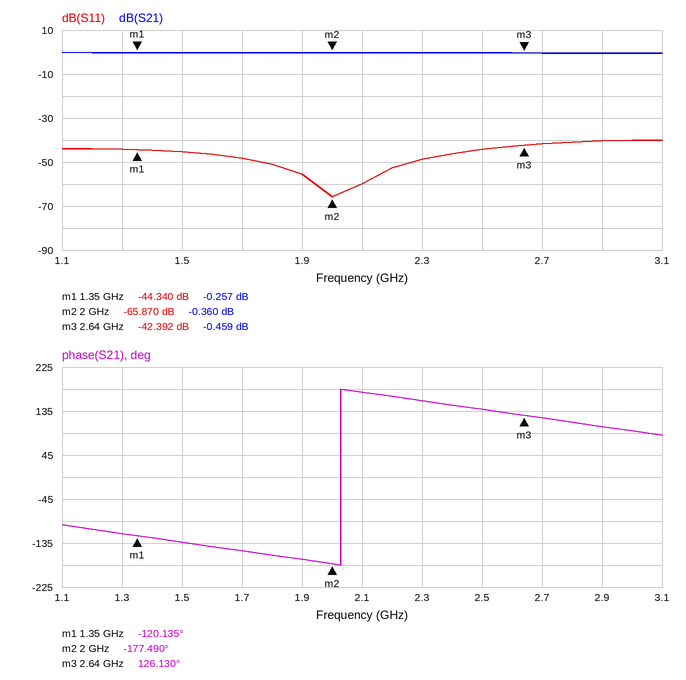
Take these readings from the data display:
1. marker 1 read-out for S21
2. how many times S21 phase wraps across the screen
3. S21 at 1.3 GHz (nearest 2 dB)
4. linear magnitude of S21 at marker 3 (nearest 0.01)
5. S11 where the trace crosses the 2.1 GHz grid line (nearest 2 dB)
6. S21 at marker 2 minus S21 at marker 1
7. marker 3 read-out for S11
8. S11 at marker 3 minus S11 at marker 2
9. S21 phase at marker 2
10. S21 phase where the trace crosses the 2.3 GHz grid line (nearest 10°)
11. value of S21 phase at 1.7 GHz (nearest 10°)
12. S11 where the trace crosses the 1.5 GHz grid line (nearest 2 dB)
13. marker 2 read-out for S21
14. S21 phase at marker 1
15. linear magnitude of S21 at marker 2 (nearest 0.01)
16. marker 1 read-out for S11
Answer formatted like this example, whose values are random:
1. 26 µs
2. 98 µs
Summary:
1. -0.257 dB
2. 1
3. 0 dB
4. 0.95
5. -60 dB
6. -0.103 dB
7. -42.392 dB
8. 23.478 dB
9. -177.490°
10. 160°
11. -150°
12. -46 dB
13. -0.360 dB
14. -120.135°
15. 0.96
16. -44.340 dB
